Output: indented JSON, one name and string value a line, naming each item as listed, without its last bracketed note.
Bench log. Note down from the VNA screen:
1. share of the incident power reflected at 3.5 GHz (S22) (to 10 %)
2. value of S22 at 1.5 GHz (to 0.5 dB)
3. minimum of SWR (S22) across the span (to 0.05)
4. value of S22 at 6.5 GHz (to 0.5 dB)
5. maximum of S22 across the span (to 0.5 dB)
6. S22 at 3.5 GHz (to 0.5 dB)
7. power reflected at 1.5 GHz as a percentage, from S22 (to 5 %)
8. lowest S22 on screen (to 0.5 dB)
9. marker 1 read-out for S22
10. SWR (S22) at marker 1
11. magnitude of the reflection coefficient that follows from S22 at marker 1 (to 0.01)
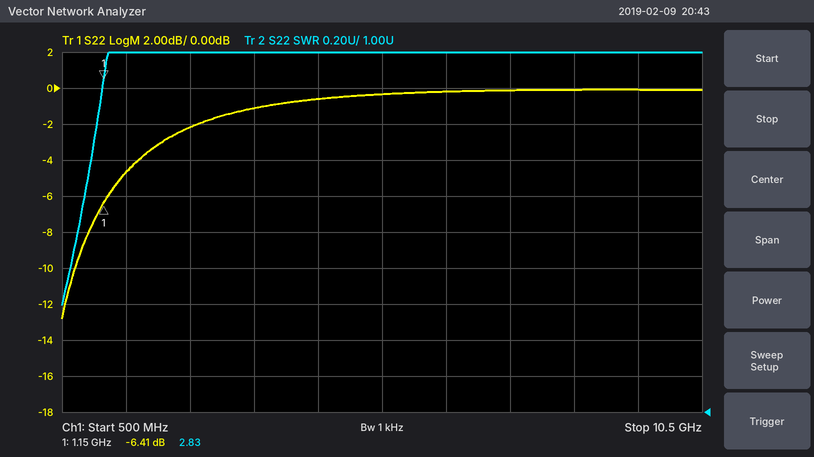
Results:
{
  "share of the incident power reflected at 3.5 GHz (S22)": "80 %",
  "value of S22 at 1.5 GHz": "-4.5 dB",
  "minimum of SWR (S22) across the span": "1.60",
  "value of S22 at 6.5 GHz": "0.0 dB",
  "maximum of S22 across the span": "0.0 dB",
  "S22 at 3.5 GHz": "-1.0 dB",
  "power reflected at 1.5 GHz as a percentage, from S22": "35 %",
  "lowest S22 on screen": "-13.0 dB",
  "marker 1 read-out for S22": "-6.41 dB",
  "SWR (S22) at marker 1": "2.83",
  "magnitude of the reflection coefficient that follows from S22 at marker 1": "0.48"
}
